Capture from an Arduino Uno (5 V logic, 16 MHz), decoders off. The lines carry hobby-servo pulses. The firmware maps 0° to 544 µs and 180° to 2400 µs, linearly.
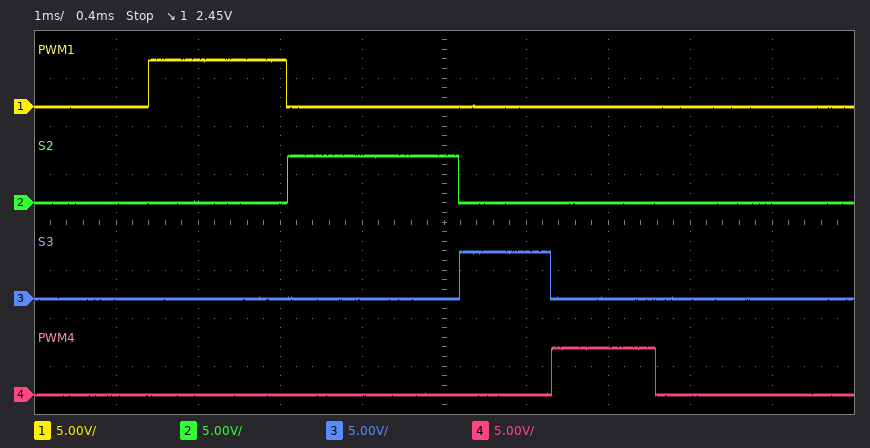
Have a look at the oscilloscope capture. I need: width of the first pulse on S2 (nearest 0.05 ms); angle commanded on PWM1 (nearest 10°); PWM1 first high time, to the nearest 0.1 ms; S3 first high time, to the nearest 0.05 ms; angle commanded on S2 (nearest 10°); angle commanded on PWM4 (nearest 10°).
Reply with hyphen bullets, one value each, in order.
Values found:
- 2.10 ms
- 110°
- 1.7 ms
- 1.10 ms
- 150°
- 70°
